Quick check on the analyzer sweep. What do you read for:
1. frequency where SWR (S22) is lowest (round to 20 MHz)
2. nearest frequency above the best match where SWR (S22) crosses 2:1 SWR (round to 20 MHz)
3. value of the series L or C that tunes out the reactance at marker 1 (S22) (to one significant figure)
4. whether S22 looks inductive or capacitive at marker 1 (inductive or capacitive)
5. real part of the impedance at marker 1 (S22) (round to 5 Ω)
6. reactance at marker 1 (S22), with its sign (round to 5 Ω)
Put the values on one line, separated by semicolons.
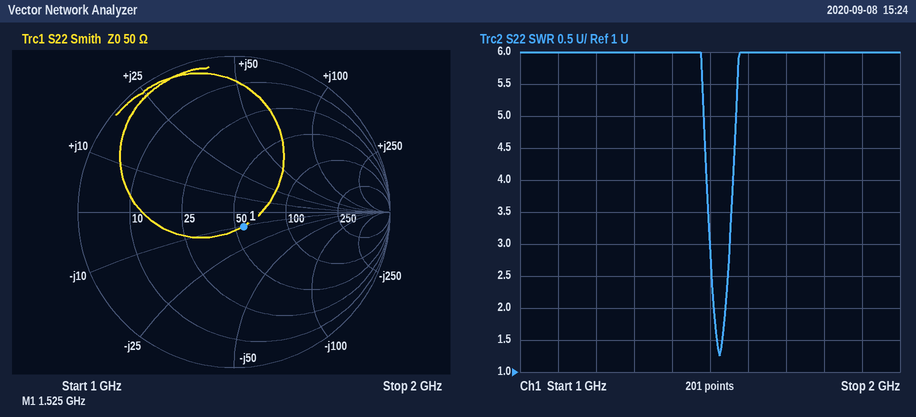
1.52 GHz; 1.54 GHz; 1 nH; capacitive; 55 Ω; -10 Ω
